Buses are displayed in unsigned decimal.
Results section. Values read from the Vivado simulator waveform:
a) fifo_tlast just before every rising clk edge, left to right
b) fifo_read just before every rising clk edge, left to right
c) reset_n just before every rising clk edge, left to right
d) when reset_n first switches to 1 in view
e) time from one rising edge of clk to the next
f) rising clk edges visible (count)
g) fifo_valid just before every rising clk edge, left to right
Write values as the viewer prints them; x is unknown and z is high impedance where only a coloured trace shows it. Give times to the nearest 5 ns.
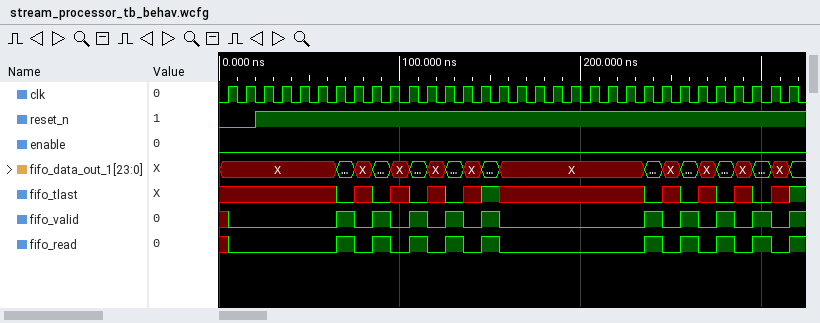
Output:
x x x x x x x 0 x 0 x 0 x 0 x 1 x x x x x x x x 0 x 0 x 0 x 0 x
x 0 0 0 0 0 0 1 0 1 0 1 0 1 0 1 0 0 0 0 0 0 0 0 1 0 1 0 1 0 1 0
0 0 1 1 1 1 1 1 1 1 1 1 1 1 1 1 1 1 1 1 1 1 1 1 1 1 1 1 1 1 1 1
20 ns
10 ns
32
x 0 0 0 0 0 0 1 0 1 0 1 0 1 0 1 0 0 0 0 0 0 0 0 1 0 1 0 1 0 1 0
